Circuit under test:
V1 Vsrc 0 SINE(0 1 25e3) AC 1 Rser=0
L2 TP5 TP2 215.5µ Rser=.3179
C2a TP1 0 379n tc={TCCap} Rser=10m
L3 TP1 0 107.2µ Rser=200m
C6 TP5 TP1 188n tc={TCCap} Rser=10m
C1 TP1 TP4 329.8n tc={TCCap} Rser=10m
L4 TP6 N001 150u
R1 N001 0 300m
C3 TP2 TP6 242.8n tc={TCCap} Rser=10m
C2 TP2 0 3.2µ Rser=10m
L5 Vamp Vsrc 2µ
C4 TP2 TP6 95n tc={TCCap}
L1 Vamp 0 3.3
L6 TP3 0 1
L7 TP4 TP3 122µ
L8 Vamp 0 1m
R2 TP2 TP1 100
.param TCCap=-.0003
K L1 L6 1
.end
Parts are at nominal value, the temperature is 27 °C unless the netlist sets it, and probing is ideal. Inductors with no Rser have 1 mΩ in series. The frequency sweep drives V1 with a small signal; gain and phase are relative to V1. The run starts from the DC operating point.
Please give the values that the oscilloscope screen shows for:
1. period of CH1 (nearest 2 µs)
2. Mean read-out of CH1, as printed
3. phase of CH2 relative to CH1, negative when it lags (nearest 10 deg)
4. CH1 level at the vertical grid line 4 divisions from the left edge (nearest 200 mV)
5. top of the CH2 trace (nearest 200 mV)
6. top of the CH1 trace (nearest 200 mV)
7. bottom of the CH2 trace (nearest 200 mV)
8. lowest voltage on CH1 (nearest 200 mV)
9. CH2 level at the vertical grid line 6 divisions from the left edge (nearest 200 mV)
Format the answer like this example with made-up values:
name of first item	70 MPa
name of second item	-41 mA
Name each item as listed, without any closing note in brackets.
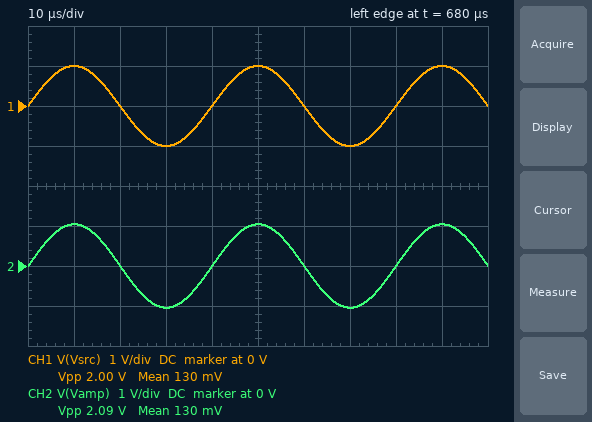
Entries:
period of CH1	40 µs
Mean read-out of CH1, as printed	130 mV
phase of CH2 relative to CH1, negative when it lags	0 deg
CH1 level at the vertical grid line 4 divisions from the left edge	0 V
top of the CH2 trace	1.0 V
top of the CH1 trace	1.0 V
bottom of the CH2 trace	-1.0 V
lowest voltage on CH1	-1.0 V
CH2 level at the vertical grid line 6 divisions from the left edge	0 V
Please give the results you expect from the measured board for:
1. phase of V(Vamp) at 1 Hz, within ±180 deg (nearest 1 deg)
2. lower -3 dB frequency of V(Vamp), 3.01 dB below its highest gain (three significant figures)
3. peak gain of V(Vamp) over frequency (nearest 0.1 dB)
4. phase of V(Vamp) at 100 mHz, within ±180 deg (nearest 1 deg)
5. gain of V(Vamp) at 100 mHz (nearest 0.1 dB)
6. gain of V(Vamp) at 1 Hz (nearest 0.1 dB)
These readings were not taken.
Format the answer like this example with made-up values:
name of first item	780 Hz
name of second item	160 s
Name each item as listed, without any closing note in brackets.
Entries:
phase of V(Vamp) at 1 Hz, within ±180 deg	9 deg
lower -3 dB frequency of V(Vamp), 3.01 dB below its highest gain	224 mHz
peak gain of V(Vamp) over frequency	0 dB
phase of V(Vamp) at 100 mHz, within ±180 deg	15 deg
gain of V(Vamp) at 100 mHz	-5.0 dB
gain of V(Vamp) at 1 Hz	-0.3 dB
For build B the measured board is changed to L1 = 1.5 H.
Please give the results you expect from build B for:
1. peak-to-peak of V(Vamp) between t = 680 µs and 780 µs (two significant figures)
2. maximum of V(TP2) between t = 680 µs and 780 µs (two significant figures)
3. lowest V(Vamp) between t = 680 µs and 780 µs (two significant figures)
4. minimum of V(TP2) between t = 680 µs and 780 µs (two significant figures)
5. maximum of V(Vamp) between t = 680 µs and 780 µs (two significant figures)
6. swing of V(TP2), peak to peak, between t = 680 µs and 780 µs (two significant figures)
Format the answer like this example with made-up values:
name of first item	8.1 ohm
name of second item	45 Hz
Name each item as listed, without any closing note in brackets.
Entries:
peak-to-peak of V(Vamp) between t = 680 µs and 780 µs	2.2 V
maximum of V(TP2) between t = 680 µs and 780 µs	1.3 V
lowest V(Vamp) between t = 680 µs and 780 µs	-1.1 V
minimum of V(TP2) between t = 680 µs and 780 µs	-1.3 V
maximum of V(Vamp) between t = 680 µs and 780 µs	1.1 V
swing of V(TP2), peak to peak, between t = 680 µs and 780 µs	2.6 V
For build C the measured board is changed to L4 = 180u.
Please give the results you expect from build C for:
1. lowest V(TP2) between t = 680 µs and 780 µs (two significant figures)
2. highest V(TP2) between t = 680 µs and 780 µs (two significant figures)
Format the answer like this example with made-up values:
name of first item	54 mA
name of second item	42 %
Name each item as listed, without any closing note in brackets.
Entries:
lowest V(TP2) between t = 680 µs and 780 µs	-850 mV
highest V(TP2) between t = 680 µs and 780 µs	850 mV
